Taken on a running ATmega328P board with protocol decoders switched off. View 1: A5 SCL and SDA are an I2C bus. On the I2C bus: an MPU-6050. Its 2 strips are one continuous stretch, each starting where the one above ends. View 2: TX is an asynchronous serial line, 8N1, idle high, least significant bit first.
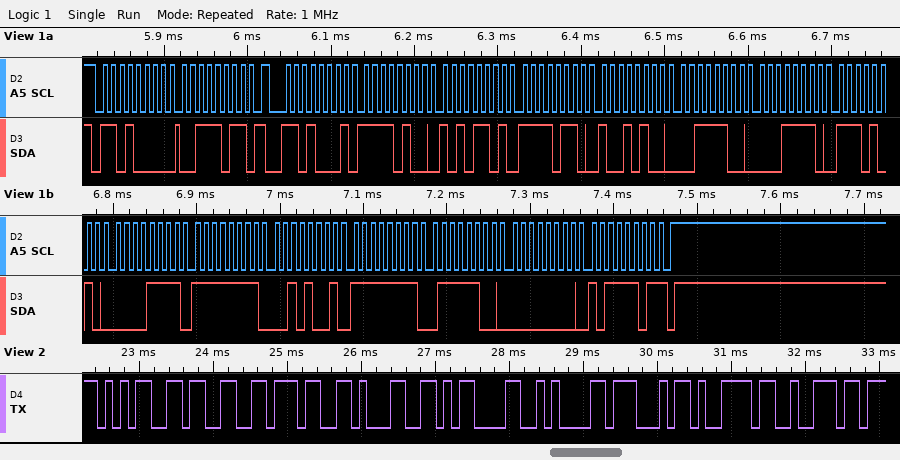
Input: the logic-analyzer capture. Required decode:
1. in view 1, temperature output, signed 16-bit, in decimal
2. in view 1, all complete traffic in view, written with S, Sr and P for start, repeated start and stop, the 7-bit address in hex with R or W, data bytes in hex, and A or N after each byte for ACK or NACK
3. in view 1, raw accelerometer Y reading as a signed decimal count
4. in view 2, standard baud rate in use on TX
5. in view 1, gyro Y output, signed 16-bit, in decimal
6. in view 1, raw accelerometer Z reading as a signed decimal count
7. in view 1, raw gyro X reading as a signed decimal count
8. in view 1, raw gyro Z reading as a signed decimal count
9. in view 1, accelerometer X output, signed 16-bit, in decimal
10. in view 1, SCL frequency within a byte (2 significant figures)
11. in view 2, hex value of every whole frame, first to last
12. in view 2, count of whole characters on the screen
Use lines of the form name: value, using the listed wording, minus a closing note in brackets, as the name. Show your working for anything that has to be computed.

in view 1, temperature output, signed 16-bit, in decimal: 0xEA0F = -5617
in view 1, all complete traffic in view, written with S, Sr and P for start, repeated start and stop, the 7-bit address in hex with R or W, data bytes in hex, and A or N after each byte for ACK or NACK: S 68W A 3B A Sr 68R A F4 A AD A F6 A 94 A 3C A 1E A EA A 0F A FF A 29 A FF A 7C A 00 A BD N P
in view 1, raw accelerometer Y reading as a signed decimal count: 0xF694 = -2412
in view 2, standard baud rate in use on TX: 9600 baud
in view 1, gyro Y output, signed 16-bit, in decimal: 0xFF7C = -132
in view 1, raw accelerometer Z reading as a signed decimal count: 0x3C1E = 15390
in view 1, raw gyro X reading as a signed decimal count: 0xFF29 = -215
in view 1, raw gyro Z reading as a signed decimal count: 0x00BD = 189
in view 1, accelerometer X output, signed 16-bit, in decimal: 0xF4AD = -2899
in view 1, SCL frequency within a byte: 100 kHz
in view 2, hex value of every whole frame, first to last: 0x35 0x33 0x37 0x31 0x0D 0x0A 0x47 0x79 0x72
in view 2, count of whole characters on the screen: 9
